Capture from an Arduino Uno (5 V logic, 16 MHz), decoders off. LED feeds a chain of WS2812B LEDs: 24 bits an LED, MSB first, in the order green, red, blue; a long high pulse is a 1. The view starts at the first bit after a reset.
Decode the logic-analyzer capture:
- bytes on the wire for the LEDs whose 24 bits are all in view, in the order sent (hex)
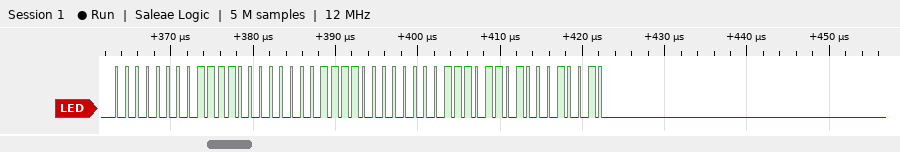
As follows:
00 F0 0F 00 ED 12
